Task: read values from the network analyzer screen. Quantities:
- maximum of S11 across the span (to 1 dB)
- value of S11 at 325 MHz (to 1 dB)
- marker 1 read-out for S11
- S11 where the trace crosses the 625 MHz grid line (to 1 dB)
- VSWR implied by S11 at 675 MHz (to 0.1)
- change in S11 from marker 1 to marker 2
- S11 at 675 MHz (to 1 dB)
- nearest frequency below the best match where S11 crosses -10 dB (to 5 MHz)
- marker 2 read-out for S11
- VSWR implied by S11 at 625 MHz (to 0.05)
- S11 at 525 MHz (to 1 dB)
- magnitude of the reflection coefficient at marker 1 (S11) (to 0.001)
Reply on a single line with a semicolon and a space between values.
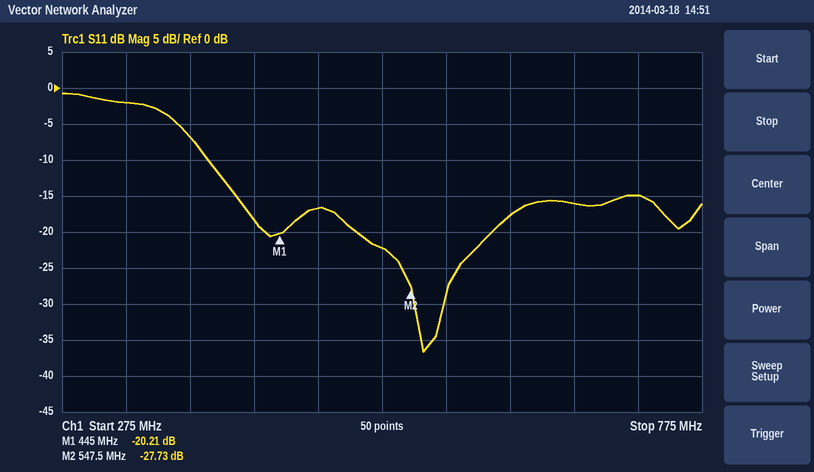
-1 dB; -2 dB; -20.21 dB; -18 dB; 1.4; -7.52 dB; -16 dB; 390 MHz; -27.73 dB; 1.30; -22 dB; 0.098
